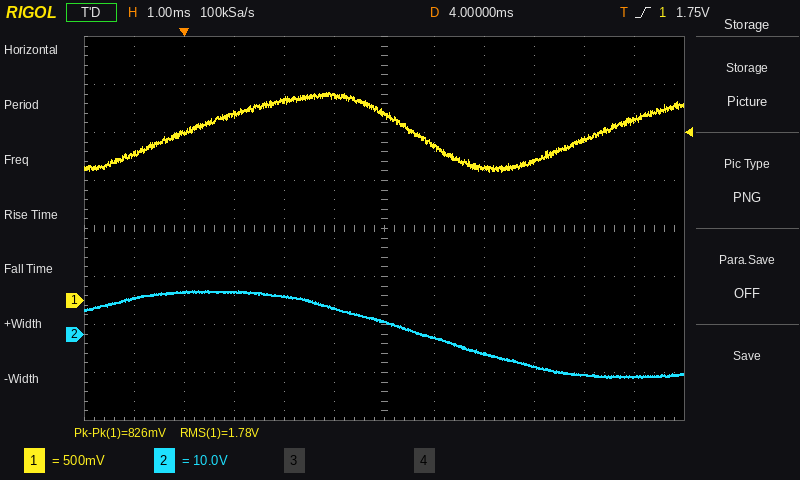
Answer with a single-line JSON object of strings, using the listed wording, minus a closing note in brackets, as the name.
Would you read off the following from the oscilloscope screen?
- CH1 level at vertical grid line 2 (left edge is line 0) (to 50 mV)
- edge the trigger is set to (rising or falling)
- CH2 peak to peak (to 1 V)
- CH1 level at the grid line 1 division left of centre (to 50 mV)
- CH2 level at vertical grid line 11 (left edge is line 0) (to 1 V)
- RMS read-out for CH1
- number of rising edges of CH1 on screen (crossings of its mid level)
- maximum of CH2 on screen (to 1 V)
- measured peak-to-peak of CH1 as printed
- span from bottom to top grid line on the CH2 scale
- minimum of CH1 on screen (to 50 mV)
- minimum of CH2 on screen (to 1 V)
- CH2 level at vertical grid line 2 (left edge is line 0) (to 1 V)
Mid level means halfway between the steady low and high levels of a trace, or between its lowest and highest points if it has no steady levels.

{"CH1 level at vertical grid line 2 (left edge is line 0)": "1.75 V", "edge the trigger is set to": "rising", "CH2 peak to peak": "18 V", "CH1 level at the grid line 1 division left of centre": "2.15 V", "CH2 level at vertical grid line 11 (left edge is line 0)": "-9 V", "RMS read-out for CH1": "1.78 V", "number of rising edges of CH1 on screen": "2", "maximum of CH2 on screen": "9 V", "measured peak-to-peak of CH1 as printed": "826 mV", "span from bottom to top grid line on the CH2 scale": "80 V", "minimum of CH1 on screen": "1.35 V", "minimum of CH2 on screen": "-9 V", "CH2 level at vertical grid line 2 (left edge is line 0)": "9 V"}
